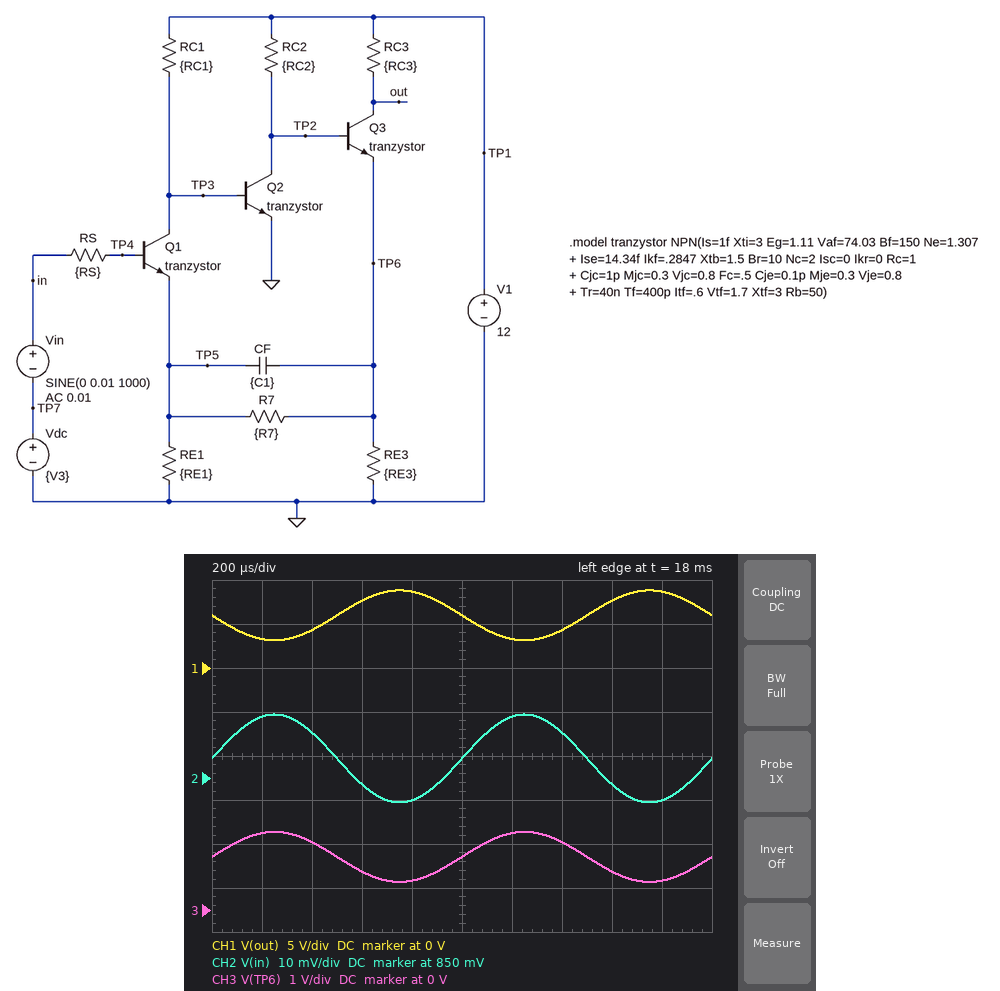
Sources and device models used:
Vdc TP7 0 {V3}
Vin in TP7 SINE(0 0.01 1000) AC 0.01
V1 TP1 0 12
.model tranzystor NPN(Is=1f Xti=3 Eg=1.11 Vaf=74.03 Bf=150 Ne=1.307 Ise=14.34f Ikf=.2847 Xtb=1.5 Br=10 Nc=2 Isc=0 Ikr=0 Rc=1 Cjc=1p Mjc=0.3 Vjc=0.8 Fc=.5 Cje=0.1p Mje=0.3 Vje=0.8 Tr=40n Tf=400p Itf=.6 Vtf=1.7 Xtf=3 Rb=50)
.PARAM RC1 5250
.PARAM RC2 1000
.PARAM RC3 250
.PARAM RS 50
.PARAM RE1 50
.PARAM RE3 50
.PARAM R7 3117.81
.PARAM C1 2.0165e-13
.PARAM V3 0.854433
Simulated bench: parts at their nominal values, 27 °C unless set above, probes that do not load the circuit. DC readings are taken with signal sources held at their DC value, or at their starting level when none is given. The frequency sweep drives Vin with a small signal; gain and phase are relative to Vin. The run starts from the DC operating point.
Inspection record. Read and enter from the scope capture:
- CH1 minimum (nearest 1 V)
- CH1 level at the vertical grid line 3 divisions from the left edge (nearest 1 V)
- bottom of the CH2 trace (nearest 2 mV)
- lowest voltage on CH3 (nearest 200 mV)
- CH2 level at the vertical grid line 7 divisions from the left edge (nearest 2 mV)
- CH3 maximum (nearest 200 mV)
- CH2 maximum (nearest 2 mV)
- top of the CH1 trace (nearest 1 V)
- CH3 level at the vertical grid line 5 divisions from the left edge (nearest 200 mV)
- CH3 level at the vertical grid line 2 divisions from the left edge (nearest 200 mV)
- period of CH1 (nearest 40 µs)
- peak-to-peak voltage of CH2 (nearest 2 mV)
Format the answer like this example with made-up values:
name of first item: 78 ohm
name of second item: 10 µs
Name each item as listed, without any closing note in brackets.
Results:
CH1 minimum: 3 V
CH1 level at the vertical grid line 3 divisions from the left edge: 8 V
bottom of the CH2 trace: 844 mV
lowest voltage on CH3: 600 mV
CH2 level at the vertical grid line 7 divisions from the left edge: 860 mV
CH3 maximum: 1.8 V
CH2 maximum: 864 mV
top of the CH1 trace: 9 V
CH3 level at the vertical grid line 5 divisions from the left edge: 1.2 V
CH3 level at the vertical grid line 2 divisions from the left edge: 1.6 V
period of CH1: 1.00 ms
peak-to-peak voltage of CH2: 20 mV
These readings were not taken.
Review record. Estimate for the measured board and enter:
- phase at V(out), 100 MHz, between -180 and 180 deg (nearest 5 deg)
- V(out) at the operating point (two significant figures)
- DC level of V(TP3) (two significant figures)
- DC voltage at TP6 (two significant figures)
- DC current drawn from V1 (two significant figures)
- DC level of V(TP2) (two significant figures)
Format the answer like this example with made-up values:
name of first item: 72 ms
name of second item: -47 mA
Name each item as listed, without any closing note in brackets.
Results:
phase at V(out), 100 MHz, between -180 and 180 deg: -20 deg
V(out) at the operating point: 6.0 V
DC level of V(TP3): 780 mV
DC voltage at TP6: 1.2 V
DC current drawn from V1: 36 mA
DC level of V(TP2): 2.0 V
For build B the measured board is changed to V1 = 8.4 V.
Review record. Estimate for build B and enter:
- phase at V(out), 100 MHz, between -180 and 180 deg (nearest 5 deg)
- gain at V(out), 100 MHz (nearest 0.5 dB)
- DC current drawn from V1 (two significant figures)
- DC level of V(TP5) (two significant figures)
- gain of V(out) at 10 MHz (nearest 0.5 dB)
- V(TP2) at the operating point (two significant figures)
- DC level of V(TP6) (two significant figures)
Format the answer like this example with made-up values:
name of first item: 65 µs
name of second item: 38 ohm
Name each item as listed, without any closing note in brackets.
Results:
phase at V(out), 100 MHz, between -180 and 180 deg: 60 deg
gain at V(out), 100 MHz: -41.5 dB
DC current drawn from V1: 34 mA
DC level of V(TP5): 110 mV
gain of V(out) at 10 MHz: -48.5 dB
V(TP2) at the operating point: 2.7 V
DC level of V(TP6): 1.6 V
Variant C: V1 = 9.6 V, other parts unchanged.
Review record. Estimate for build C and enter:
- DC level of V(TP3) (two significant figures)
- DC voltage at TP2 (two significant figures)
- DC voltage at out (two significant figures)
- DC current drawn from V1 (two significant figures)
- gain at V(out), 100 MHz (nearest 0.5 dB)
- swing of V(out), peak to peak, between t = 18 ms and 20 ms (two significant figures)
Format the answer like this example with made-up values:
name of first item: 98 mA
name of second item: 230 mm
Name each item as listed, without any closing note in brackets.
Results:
DC level of V(TP3): 240 mV
DC voltage at TP2: 3.0 V
DC voltage at out: 1.9 V
DC current drawn from V1: 39 mA
gain at V(out), 100 MHz: -41.5 dB
swing of V(out), peak to peak, between t = 18 ms and 20 ms: 44 mV
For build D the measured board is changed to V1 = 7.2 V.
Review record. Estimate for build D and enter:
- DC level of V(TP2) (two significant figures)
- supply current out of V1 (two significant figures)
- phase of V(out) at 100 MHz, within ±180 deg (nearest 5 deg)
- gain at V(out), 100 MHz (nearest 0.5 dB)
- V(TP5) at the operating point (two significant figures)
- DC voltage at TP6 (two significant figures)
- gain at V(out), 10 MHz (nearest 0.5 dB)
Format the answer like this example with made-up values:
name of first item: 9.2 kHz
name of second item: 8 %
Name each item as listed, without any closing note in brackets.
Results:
DC level of V(TP2): 2.4 V
supply current out of V1: 29 mA
phase of V(out) at 100 MHz, within ±180 deg: 60 deg
gain at V(out), 100 MHz: -41.5 dB
V(TP5) at the operating point: 97 mV
DC voltage at TP6: 1.4 V
gain at V(out), 10 MHz: -48.0 dB
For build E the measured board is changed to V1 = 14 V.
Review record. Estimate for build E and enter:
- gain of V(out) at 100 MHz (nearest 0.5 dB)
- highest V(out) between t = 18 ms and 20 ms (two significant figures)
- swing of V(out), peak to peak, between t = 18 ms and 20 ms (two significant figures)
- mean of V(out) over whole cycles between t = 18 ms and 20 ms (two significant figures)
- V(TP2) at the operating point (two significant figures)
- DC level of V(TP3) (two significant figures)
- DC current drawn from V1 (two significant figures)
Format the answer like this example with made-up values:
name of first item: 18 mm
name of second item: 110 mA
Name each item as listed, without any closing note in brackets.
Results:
gain of V(out) at 100 MHz: -35.5 dB
highest V(out) between t = 18 ms and 20 ms: 14 V
swing of V(out), peak to peak, between t = 18 ms and 20 ms: 2.5 V
mean of V(out) over whole cycles between t = 18 ms and 20 ms: 13 V
V(TP2) at the operating point: 160 mV
DC level of V(TP3): 800 mV
DC current drawn from V1: 16 mA
